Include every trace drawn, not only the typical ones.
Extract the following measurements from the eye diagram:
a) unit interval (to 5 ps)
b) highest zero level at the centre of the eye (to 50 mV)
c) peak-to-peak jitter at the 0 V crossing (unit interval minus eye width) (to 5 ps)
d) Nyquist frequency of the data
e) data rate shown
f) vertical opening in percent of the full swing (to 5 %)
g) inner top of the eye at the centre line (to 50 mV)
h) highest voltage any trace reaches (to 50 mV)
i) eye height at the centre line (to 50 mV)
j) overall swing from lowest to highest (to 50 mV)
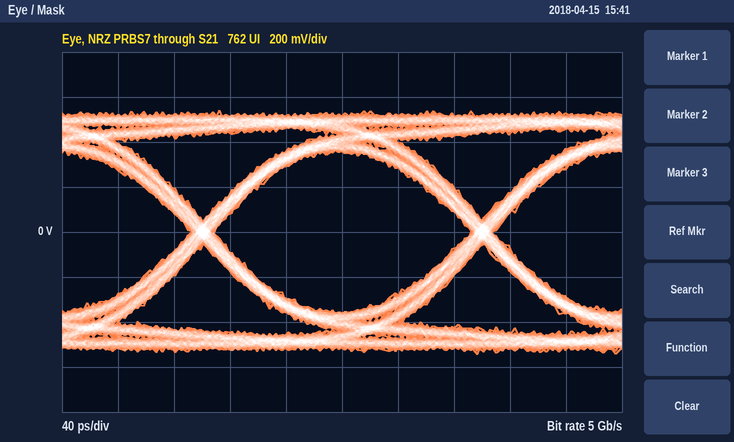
200 ps
-350 mV
15 ps
2.5 GHz
5 Gb/s
65 %
350 mV
550 mV
700 mV
1.10 V
